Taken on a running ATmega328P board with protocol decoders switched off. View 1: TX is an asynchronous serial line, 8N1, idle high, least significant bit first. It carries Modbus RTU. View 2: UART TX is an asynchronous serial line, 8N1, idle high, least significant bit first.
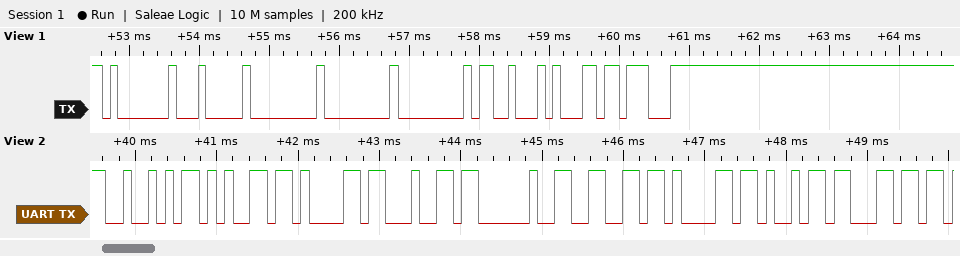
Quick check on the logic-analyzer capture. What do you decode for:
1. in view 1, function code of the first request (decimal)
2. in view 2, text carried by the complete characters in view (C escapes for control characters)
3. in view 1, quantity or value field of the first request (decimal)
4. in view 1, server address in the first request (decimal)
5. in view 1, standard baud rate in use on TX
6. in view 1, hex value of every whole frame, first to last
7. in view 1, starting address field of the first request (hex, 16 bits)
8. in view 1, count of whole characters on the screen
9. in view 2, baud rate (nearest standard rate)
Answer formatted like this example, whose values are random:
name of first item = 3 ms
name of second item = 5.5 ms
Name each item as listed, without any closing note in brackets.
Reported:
in view 1, function code of the first request = 4
in view 2, text carried by the complete characters in view = "Read fail"
in view 1, quantity or value field of the first request = 19
in view 1, server address in the first request = 1
in view 1, standard baud rate in use on TX = 9600 baud
in view 1, hex value of every whole frame, first to last = 01 04 00 00 00 13 B1 C7
in view 1, starting address field of the first request = 0x0000
in view 1, count of whole characters on the screen = 8
in view 2, baud rate = 9600 baud
